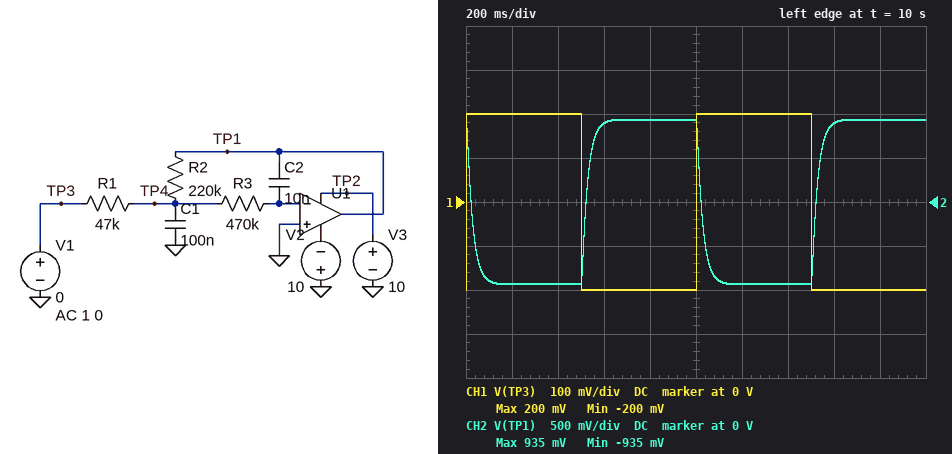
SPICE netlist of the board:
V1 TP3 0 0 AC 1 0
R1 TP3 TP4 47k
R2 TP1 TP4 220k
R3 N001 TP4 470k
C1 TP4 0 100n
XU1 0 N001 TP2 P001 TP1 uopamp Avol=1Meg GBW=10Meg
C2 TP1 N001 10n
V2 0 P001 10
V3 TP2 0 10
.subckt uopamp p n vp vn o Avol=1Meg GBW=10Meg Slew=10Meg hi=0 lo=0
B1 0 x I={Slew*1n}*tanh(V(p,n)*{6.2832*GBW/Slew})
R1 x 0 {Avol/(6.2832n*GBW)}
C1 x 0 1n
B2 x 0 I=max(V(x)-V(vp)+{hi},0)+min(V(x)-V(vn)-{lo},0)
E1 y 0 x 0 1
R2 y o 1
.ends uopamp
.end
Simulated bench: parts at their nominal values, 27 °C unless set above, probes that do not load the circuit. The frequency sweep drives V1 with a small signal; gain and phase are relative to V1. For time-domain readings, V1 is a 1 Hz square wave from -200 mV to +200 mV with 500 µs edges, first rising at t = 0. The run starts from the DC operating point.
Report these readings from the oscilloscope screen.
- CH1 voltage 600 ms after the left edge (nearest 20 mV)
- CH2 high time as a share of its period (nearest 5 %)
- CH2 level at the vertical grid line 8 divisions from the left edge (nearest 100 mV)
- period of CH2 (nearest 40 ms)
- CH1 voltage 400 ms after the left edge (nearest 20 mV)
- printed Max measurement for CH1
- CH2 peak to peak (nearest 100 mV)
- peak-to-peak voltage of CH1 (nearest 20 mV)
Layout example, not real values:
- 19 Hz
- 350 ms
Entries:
- -200 mV
- 50 %
- 900 mV
- 1.00 s
- 200 mV
- 200 mV
- 1.9 V
- 400 mV
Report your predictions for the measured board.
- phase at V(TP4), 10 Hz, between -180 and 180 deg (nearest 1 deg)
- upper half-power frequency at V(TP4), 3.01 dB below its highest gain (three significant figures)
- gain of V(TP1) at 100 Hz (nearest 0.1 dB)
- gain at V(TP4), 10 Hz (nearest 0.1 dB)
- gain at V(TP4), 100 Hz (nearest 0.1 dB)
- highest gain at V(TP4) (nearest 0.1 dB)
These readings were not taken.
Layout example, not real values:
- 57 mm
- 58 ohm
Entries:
- 18 deg
- 49.4 Hz
- -19.4 dB
- -2.8 dB
- -10.0 dB
- -2.4 dB
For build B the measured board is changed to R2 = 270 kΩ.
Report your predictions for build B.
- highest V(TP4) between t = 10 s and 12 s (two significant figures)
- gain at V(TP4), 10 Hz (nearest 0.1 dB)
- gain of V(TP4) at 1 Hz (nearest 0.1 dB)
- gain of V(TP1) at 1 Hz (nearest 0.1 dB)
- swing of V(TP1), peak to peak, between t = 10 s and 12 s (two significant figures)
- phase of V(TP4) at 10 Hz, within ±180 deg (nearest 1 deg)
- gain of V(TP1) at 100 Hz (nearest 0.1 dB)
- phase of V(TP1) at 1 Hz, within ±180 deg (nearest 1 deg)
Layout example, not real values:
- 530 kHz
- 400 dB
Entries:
- 260 mV
- -2.3 dB
- -15.6 dB
- 15.0 dB
- 2.3 V
- 13 deg
- -19.4 dB
- 168 deg
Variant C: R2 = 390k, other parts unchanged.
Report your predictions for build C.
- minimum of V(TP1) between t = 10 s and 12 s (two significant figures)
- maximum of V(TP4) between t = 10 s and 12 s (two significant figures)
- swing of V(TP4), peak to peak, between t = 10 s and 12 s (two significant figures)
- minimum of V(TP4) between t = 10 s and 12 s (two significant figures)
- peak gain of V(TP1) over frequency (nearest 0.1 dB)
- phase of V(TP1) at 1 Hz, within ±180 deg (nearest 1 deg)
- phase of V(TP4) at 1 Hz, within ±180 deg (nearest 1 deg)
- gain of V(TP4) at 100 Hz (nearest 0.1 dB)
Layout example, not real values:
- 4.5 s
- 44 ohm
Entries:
- -1.7 V
- 280 mV
- 560 mV
- -280 mV
- 18.4 dB
- 163 deg
- 73 deg
- -10.0 dB
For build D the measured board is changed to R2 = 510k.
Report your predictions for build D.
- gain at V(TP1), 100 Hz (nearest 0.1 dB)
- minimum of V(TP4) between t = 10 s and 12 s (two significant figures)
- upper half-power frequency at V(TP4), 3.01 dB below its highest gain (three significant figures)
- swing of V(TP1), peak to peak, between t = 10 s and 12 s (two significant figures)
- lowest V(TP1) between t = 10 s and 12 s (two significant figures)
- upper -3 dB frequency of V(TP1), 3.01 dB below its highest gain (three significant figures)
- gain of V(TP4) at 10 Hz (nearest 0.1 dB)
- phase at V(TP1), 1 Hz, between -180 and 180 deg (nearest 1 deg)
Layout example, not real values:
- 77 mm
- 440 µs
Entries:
- -19.4 dB
- -290 mV
- 42.8 Hz
- 4.3 V
- -2.2 V
- 2.80 Hz
- -1.5 dB
- 159 deg
